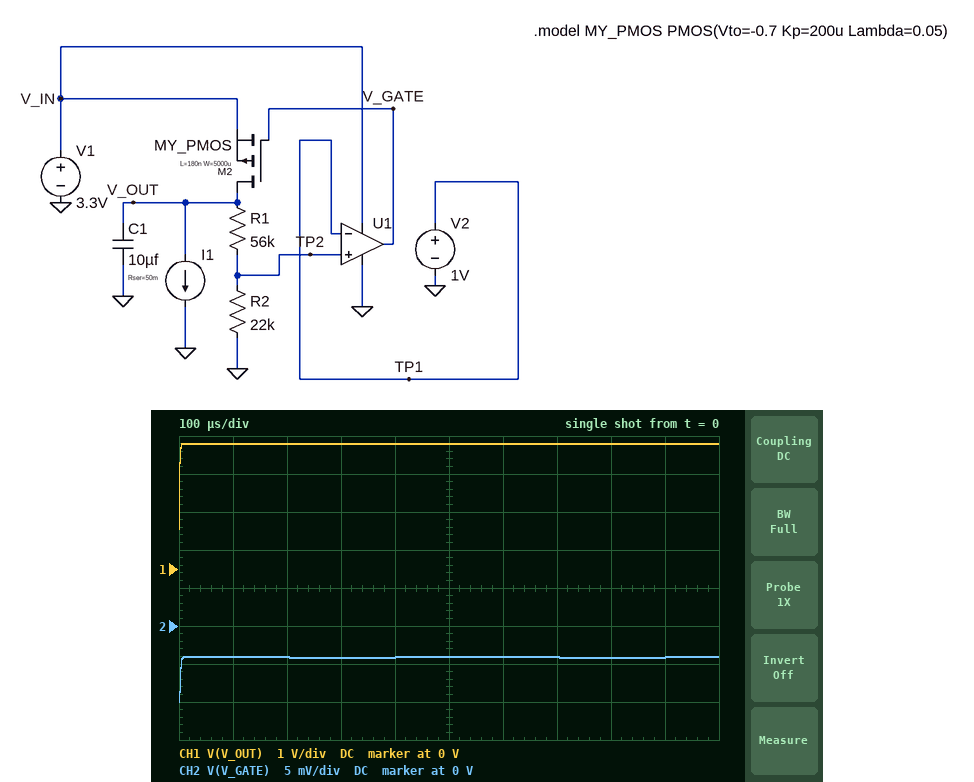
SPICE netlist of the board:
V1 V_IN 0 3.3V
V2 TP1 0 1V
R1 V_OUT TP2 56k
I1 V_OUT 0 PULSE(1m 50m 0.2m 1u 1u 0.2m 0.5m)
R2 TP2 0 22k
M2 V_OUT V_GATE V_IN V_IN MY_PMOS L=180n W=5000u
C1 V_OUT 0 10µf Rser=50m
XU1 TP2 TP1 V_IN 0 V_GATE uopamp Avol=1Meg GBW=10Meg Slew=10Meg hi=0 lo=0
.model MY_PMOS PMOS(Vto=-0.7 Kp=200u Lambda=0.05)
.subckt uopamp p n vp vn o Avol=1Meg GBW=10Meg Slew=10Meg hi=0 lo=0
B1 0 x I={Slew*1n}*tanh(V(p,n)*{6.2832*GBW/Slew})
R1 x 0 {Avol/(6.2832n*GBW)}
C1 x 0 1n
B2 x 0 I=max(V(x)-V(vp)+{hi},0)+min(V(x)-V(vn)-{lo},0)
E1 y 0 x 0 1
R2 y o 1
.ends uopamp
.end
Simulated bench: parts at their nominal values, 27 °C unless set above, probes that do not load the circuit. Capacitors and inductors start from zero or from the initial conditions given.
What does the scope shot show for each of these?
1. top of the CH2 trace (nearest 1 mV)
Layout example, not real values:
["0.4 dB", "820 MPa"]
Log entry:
["-4 mV"]
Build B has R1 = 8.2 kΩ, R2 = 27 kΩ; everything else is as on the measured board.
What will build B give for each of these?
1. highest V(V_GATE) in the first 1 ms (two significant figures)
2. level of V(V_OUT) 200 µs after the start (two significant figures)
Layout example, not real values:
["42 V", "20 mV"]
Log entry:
["3.3 V", "1.3 V"]
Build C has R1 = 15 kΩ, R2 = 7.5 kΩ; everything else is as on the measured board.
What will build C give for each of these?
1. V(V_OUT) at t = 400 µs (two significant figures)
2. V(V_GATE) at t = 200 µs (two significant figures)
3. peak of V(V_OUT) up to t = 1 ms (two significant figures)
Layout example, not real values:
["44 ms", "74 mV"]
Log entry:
["3.0 V", "3.3 V", "3.1 V"]
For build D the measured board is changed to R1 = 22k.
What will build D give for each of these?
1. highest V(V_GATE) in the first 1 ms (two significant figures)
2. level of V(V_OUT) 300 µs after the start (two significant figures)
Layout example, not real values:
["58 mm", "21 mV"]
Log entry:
["3.3 V", "2.0 V"]
